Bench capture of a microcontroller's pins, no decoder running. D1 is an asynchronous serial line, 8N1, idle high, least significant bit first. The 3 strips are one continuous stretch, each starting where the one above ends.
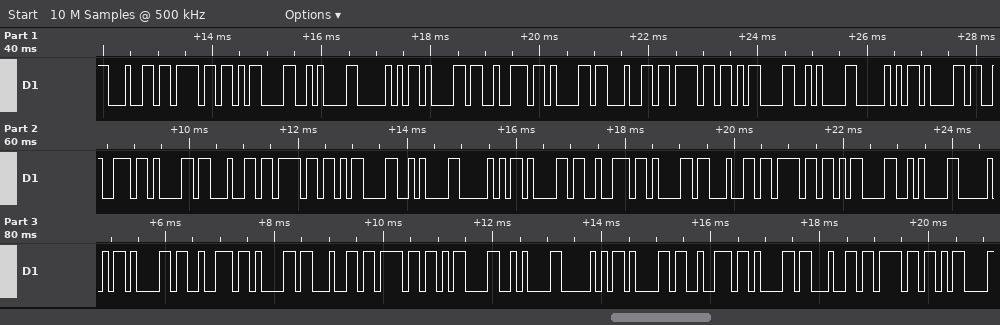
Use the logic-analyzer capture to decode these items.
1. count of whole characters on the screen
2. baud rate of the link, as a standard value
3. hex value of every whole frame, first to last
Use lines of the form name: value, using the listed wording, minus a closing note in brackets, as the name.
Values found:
count of whole characters on the screen: 43
baud rate of the link, as a standard value: 9600 baud
hex value of every whole frame, first to last: 0x64 0x6F 0x0D 0x0A 0x50 0x61 0x72 0x61 0x64 0x6F 0x0D 0x0A 0x50 0x61 0x72 0x61 0x64 0x6F 0x0D 0x0A 0x50 0x61 0x72 0x61 0x64 0x6F 0x0D 0x0A 0x50 0x61 0x72 0x61 0x64 0x6F 0x0D 0x0A 0x50 0x61 0x72 0x61 0x64 0x6F 0x0D
